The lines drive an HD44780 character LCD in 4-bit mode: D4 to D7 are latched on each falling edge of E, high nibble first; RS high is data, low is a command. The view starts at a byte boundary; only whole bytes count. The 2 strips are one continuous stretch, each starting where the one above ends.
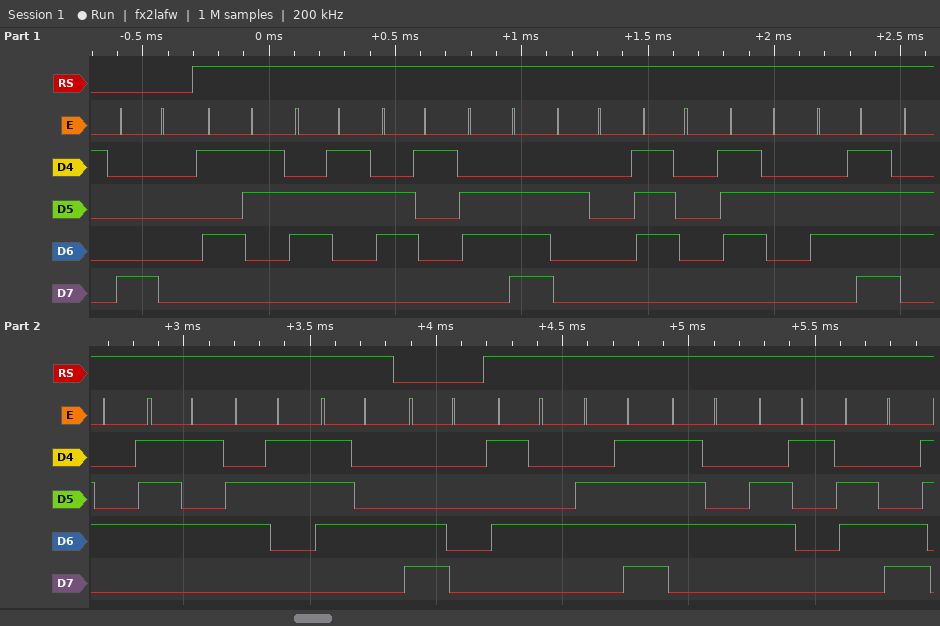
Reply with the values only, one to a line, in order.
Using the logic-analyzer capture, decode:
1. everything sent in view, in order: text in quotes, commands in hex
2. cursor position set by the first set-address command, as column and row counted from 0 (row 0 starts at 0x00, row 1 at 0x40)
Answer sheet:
0x80 "Scan product" 0xC0 "Total"
column 0, row 0
